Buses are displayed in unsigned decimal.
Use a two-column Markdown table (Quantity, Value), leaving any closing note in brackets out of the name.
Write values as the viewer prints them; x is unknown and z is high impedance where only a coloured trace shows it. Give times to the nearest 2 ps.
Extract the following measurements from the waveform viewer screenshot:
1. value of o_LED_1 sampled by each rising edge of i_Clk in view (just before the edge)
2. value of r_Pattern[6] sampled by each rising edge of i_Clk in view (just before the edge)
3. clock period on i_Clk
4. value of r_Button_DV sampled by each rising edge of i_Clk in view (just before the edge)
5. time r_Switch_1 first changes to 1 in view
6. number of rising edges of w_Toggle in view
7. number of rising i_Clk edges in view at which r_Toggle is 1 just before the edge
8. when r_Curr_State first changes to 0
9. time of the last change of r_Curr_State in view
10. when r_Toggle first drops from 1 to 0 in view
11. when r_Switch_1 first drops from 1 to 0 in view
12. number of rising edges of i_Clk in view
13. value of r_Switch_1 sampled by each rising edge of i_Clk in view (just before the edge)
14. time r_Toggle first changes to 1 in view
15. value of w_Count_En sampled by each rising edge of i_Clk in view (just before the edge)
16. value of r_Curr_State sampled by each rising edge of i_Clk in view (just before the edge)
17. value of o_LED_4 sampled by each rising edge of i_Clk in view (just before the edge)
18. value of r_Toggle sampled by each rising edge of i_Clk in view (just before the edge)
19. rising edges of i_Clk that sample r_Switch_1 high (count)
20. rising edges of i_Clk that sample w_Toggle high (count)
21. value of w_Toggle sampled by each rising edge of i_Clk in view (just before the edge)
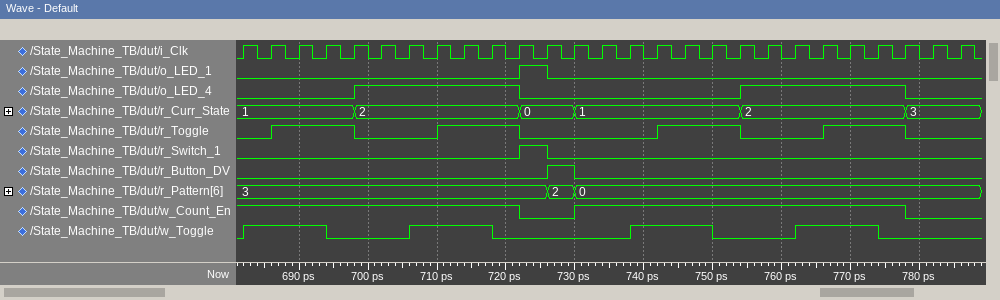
| Quantity | Value |
|---|---|
| value of o_LED_1 sampled by each rising edge of i_Clk in view | 0 0 0 0 0 0 0 0 0 0 0 1 0 0 0 0 0 0 0 0 0 0 0 0 0 0 0 |
| value of r_Pattern[6] sampled by each rising edge of i_Clk in view | 3, 3, 3, 3, 3, 3, 3, 3, 3, 3, 3, 3, 2, 0, 0, 0, 0, 0, 0, 0, 0, 0, 0, 0, 0, 0, 0 |
| clock period on i_Clk | 4 ps |
| value of r_Button_DV sampled by each rising edge of i_Clk in view | 0 0 0 0 0 0 0 0 0 0 0 0 1 0 0 0 0 0 0 0 0 0 0 0 0 0 0 |
| time r_Switch_1 first changes to 1 in view | 722 ps |
| number of rising edges of w_Toggle in view | 4 |
| number of rising i_Clk edges in view at which r_Toggle is 1 just before the edge | 12 |
| when r_Curr_State first changes to 0 | 722 ps |
| time of the last change of r_Curr_State in view | 778 ps |
| when r_Toggle first drops from 1 to 0 in view | 698 ps |
| when r_Switch_1 first drops from 1 to 0 in view | 726 ps |
| number of rising edges of i_Clk in view | 27 |
| value of r_Switch_1 sampled by each rising edge of i_Clk in view | 0 0 0 0 0 0 0 0 0 0 0 1 0 0 0 0 0 0 0 0 0 0 0 0 0 0 0 |
| time r_Toggle first changes to 1 in view | 686 ps |
| value of w_Count_En sampled by each rising edge of i_Clk in view | 1 1 1 1 1 1 1 1 1 1 1 0 0 1 1 1 1 1 1 1 1 1 1 1 1 0 0 |
| value of r_Curr_State sampled by each rising edge of i_Clk in view | 1, 1, 1, 1, 1, 2, 2, 2, 2, 2, 2, 0, 0, 1, 1, 1, 1, 1, 1, 2, 2, 2, 2, 2, 2, 3, 3 |
| value of o_LED_4 sampled by each rising edge of i_Clk in view | 0 0 0 0 0 1 1 1 1 1 1 0 0 0 0 0 0 0 0 1 1 1 1 1 1 0 0 |
| value of r_Toggle sampled by each rising edge of i_Clk in view | 0 0 1 1 1 0 0 0 1 1 1 0 0 0 0 0 1 1 1 0 0 0 1 1 1 0 0 |
| rising edges of i_Clk that sample r_Switch_1 high | 1 |
| rising edges of i_Clk that sample w_Toggle high | 12 |
| value of w_Toggle sampled by each rising edge of i_Clk in view | 0 1 1 1 0 0 0 1 1 1 0 0 0 0 0 1 1 1 0 0 0 1 1 1 0 0 0 |
